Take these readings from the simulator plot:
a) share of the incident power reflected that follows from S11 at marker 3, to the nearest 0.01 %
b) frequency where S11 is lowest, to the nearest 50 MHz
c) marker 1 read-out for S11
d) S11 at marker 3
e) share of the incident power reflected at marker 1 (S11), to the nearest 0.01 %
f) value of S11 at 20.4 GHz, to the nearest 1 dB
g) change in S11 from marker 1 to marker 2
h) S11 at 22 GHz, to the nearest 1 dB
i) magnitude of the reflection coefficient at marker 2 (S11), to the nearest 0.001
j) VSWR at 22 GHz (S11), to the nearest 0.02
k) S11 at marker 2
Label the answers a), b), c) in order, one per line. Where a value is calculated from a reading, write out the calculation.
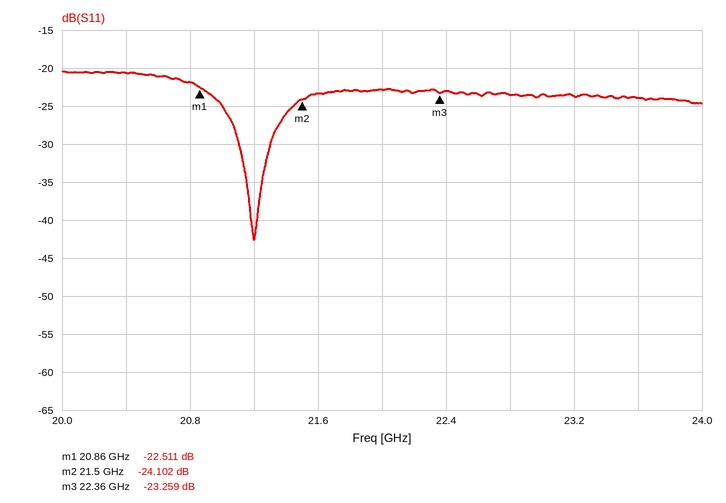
a) 10^(-23.259/10) ≈ 0.47 %
b) 21.20 GHz
c) -22.511 dB
d) -23.259 dB
e) 10^(-22.511/10) ≈ 0.56 %
f) -21 dB
g) -24.102 − (-22.511) = -1.591 dB
h) -23 dB
i) 10^(-24.102/20) ≈ 0.062
j) |Γ| = 10^(-23/20) = 0.0708; VSWR = (1 + 0.0708)/(1 − 0.0708) ≈ 1.15, so 1.16 to the nearest 0.02
k) -24.102 dB
